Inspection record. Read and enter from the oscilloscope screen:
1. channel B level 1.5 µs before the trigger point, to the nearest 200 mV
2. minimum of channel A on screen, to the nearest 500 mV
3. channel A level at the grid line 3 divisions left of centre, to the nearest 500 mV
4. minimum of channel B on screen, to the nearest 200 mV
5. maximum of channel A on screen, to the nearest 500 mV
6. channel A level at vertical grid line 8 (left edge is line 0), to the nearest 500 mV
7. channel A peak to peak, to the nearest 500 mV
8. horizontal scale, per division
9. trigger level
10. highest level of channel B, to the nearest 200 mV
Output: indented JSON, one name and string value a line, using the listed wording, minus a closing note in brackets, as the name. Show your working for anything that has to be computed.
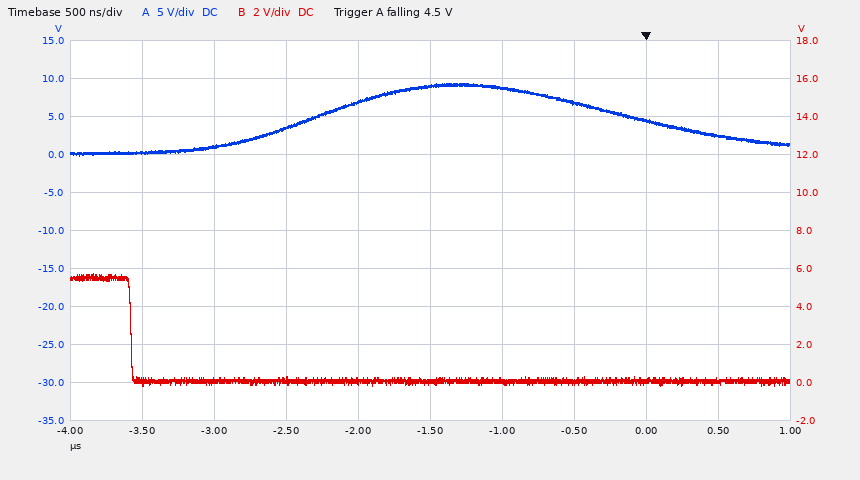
{
  "channel B level 1.5 µs before the trigger point, to the nearest 200 mV": "0.0 V",
  "minimum of channel A on screen, to the nearest 500 mV": "0.0 V",
  "channel A level at the grid line 3 divisions left of centre, to the nearest 500 mV": "1.0 V",
  "minimum of channel B on screen, to the nearest 200 mV": "-200 mV",
  "maximum of channel A on screen, to the nearest 500 mV": "9.5 V",
  "channel A level at vertical grid line 8 (left edge is line 0), to the nearest 500 mV": "4.5 V",
  "channel A peak to peak, to the nearest 500 mV": "9.5 V − (0.0 V) = 9.5 V",
  "horizontal scale, per division": "500 ns",
  "trigger level": "4.5 V",
  "highest level of channel B, to the nearest 200 mV": "5.8 V"
}
